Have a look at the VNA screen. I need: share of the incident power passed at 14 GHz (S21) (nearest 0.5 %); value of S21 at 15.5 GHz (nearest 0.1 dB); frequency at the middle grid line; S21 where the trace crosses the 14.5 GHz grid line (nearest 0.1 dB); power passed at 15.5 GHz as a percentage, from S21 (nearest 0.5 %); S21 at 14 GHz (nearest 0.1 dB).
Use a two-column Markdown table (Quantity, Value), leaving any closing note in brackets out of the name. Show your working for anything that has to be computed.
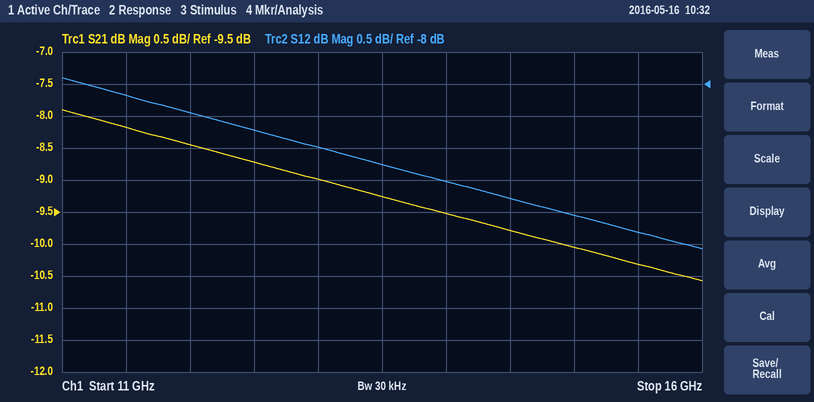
| Quantity | Value |
|---|---|
| share of the incident power passed at 14 GHz (S21) | 10^(-9.5/10) ≈ 11.2 %, so 11.0 % to the nearest 0.5 % |
| value of S21 at 15.5 GHz | -10.3 dB |
| frequency at the middle grid line | 13.5 GHz |
| S21 where the trace crosses the 14.5 GHz grid line | -9.8 dB |
| power passed at 15.5 GHz as a percentage, from S21 | 10^(-10.3/10) ≈ 9.33 %, so 9.5 % to the nearest 0.5 % |
| S21 at 14 GHz | -9.5 dB |
